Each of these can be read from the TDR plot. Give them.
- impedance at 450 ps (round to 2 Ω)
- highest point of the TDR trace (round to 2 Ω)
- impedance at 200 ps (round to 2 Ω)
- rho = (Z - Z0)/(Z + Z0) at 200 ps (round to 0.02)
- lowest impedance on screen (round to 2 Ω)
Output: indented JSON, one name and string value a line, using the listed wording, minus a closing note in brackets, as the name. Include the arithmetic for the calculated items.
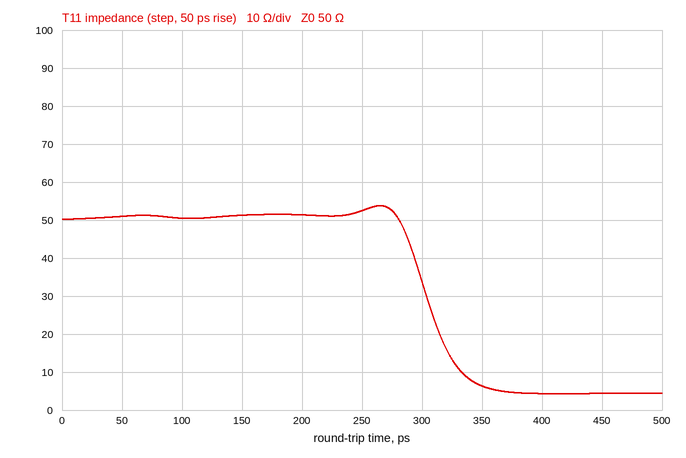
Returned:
{
  "impedance at 450 ps": "4 Ω",
  "highest point of the TDR trace": "54 Ω",
  "impedance at 200 ps": "52 Ω",
  "rho = (Z - Z0)/(Z + Z0) at 200 ps": "(52 − 50)/(52 + 50) ≈ +0.02",
  "lowest impedance on screen": "4 Ω"
}
